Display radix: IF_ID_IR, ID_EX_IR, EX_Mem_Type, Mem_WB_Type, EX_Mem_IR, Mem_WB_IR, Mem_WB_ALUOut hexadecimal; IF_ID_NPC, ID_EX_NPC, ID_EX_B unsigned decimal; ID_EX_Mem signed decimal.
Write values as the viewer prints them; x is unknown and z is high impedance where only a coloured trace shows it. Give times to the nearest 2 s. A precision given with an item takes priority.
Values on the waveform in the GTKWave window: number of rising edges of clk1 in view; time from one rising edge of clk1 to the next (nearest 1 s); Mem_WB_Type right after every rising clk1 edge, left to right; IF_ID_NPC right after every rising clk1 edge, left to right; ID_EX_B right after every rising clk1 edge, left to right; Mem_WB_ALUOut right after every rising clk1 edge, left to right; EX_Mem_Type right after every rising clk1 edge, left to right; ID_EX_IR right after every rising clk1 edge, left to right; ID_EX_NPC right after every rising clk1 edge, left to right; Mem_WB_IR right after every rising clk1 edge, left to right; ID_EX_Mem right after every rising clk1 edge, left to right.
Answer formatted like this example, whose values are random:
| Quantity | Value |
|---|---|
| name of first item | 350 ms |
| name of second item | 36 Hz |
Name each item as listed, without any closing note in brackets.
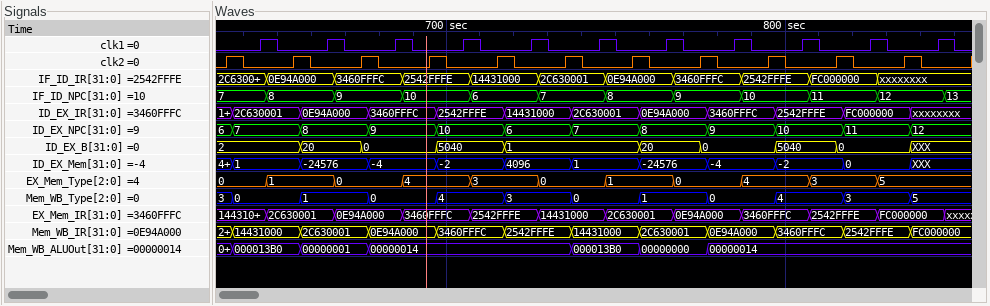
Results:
| Quantity | Value |
|---|---|
| number of rising edges of clk1 in view | 11 |
| time from one rising edge of clk1 to the next | 20 s |
| Mem_WB_Type right after every rising clk1 edge, left to right | 0, 1, 0, 4, 3, 0, 1, 0, 4, 3, 5 |
| IF_ID_NPC right after every rising clk1 edge, left to right | 7, 8, 9, 10, 6, 7, 8, 9, 10, 11, 12 |
| ID_EX_B right after every rising clk1 edge, left to right | 2, 20, 0, 5040, 1, 1, 20, 0, 5040, 0, XXX |
| Mem_WB_ALUOut right after every rising clk1 edge, left to right | 000013B0, 00000001, 00000014, 00000014, 00000014, 000013B0, 00000000, 00000014, 00000014, 00000014, 00000014 |
| EX_Mem_Type right after every rising clk1 edge, left to right | 0, 1, 0, 4, 3, 0, 1, 0, 4, 3, 5 |
| ID_EX_IR right after every rising clk1 edge, left to right | 2C630001, 0E94A000, 3460FFFC, 2542FFFE, 14431000, 2C630001, 0E94A000, 3460FFFC, 2542FFFE, FC000000, xxxxxxxx |
| ID_EX_NPC right after every rising clk1 edge, left to right | 7, 8, 9, 10, 6, 7, 8, 9, 10, 11, 12 |
| Mem_WB_IR right after every rising clk1 edge, left to right | 14431000, 2C630001, 0E94A000, 3460FFFC, 2542FFFE, 14431000, 2C630001, 0E94A000, 3460FFFC, 2542FFFE, FC000000 |
| ID_EX_Mem right after every rising clk1 edge, left to right | 1, -24576, -4, -2, 4096, 1, -24576, -4, -2, 0, XXX |
